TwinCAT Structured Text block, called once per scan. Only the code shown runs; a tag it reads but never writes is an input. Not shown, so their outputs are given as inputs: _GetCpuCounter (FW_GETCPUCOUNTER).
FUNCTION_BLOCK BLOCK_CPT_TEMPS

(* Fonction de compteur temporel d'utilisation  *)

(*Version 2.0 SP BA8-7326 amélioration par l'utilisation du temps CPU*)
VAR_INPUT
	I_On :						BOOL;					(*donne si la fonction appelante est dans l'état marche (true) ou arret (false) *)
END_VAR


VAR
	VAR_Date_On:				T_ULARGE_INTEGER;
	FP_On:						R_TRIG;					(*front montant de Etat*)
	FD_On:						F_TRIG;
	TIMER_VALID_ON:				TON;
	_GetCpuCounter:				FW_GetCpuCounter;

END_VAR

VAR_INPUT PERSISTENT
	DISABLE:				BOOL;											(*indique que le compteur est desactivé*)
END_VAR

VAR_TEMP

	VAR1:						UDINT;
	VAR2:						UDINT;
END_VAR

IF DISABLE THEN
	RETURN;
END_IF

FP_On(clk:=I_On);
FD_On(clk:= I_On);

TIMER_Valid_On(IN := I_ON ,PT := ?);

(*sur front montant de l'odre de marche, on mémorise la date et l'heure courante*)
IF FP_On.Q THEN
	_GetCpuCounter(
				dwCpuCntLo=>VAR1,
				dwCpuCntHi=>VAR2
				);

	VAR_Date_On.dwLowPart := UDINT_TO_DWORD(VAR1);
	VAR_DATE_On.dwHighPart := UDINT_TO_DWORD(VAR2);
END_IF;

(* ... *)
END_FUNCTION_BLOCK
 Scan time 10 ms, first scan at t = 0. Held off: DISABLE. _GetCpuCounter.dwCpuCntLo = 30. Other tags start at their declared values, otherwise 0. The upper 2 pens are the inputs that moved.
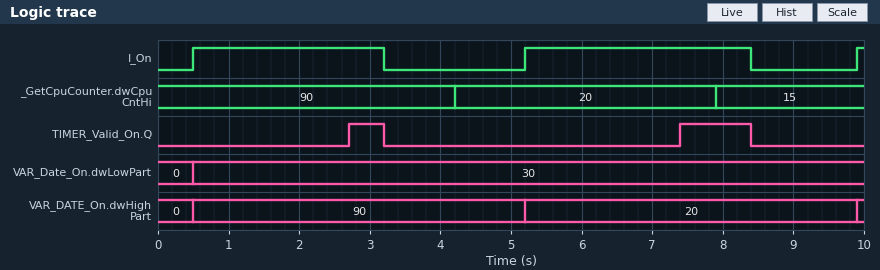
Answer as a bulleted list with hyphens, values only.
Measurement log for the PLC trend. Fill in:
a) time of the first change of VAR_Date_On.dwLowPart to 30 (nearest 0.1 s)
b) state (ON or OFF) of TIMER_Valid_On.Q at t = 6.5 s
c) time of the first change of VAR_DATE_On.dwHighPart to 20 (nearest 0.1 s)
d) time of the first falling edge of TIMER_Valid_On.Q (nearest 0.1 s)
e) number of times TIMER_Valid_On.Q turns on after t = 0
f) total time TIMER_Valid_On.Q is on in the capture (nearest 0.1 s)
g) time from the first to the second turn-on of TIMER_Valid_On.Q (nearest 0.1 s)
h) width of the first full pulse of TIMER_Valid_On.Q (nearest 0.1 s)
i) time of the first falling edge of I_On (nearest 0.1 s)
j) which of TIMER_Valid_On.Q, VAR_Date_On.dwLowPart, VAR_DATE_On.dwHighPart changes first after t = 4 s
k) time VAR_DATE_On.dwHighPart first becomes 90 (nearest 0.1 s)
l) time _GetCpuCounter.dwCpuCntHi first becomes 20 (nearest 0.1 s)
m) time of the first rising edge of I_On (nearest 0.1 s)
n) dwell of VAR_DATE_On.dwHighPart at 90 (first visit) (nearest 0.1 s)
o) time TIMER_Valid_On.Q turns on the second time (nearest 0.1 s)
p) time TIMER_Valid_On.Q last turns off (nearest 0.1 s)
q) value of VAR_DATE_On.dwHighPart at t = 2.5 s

- 0.5 s
- OFF
- 5.2 s
- 3.2 s
- 2
- 1.5 s
- 4.7 s
- 0.5 s
- 3.2 s
- VAR_DATE_On.dwHighPart
- 0.5 s
- 4.2 s
- 0.5 s
- 4.7 s
- 7.4 s
- 8.4 s
- 90
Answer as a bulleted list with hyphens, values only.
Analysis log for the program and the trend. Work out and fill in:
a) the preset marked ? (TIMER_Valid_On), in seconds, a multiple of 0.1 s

- 2.2 s
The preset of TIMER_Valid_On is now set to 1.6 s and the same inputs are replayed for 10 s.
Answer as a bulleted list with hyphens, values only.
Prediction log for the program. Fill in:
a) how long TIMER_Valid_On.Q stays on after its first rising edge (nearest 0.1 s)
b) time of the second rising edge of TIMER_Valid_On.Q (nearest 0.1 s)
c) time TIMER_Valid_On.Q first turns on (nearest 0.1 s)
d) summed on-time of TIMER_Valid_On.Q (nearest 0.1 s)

- 1.1 s
- 6.8 s
- 2.1 s
- 2.7 s
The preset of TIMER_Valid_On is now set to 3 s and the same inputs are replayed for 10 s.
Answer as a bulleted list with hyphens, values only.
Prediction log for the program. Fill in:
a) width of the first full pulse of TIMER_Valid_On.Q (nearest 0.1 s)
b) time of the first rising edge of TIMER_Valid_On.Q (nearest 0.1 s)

- 0.2 s
- 8.2 s
